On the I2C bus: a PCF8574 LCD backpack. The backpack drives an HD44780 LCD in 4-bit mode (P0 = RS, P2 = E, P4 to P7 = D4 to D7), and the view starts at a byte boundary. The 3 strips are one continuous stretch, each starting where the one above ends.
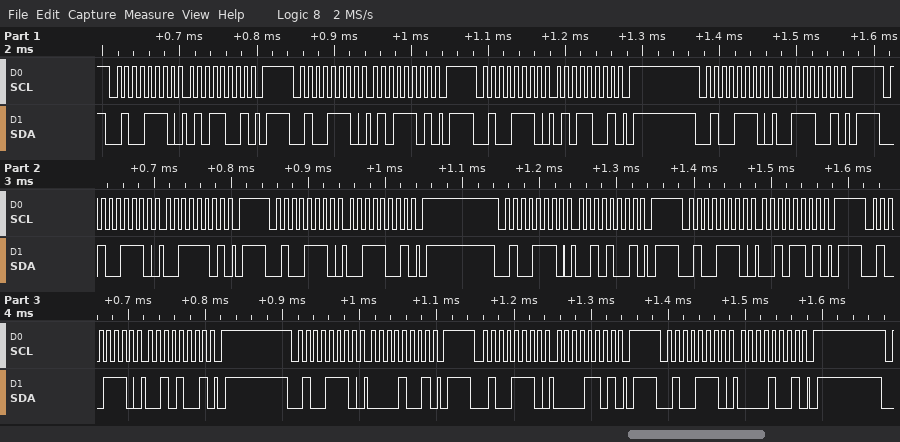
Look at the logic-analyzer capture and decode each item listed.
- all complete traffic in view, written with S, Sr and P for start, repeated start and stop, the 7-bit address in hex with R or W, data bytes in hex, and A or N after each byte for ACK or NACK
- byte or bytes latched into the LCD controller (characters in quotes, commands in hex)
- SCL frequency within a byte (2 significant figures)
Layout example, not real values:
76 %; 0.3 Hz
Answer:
S 27W A 59 A P S 27W A 5D A P S 27W A 59 A P S 27W A 39 A P S 27W A 3D A P S 27W A 39 A P S 27W A 29 A P S 27W A 2D A P S 27W A 29 A P S 27W A 09 A P S 27W A 0D A P S 27W A 09 A P; 'S' ' '; 100 kHz
